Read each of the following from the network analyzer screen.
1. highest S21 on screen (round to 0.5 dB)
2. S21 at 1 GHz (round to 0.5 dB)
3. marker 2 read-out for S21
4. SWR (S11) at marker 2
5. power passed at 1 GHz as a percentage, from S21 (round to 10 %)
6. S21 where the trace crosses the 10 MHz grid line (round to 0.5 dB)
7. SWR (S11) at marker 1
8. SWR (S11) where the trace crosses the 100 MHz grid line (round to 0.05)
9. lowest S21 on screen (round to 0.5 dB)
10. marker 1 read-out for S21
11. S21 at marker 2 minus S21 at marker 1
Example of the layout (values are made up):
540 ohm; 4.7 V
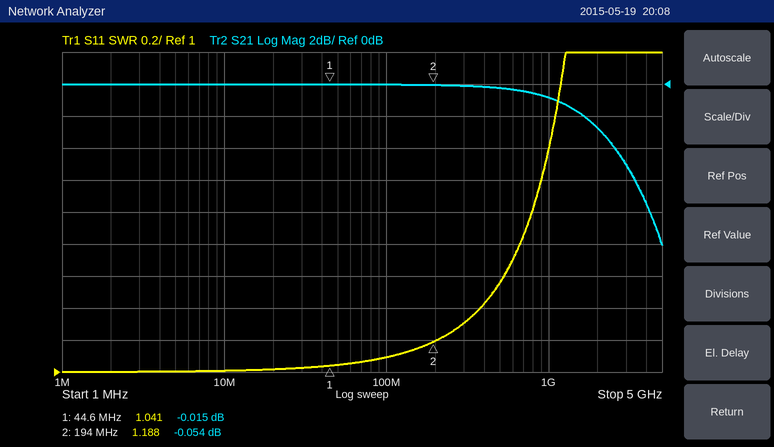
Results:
0.0 dB; -1.0 dB; -0.054 dB; 1.188; 80 %; 0.0 dB; 1.041; 1.10; -10.0 dB; -0.015 dB; -0.039 dB
